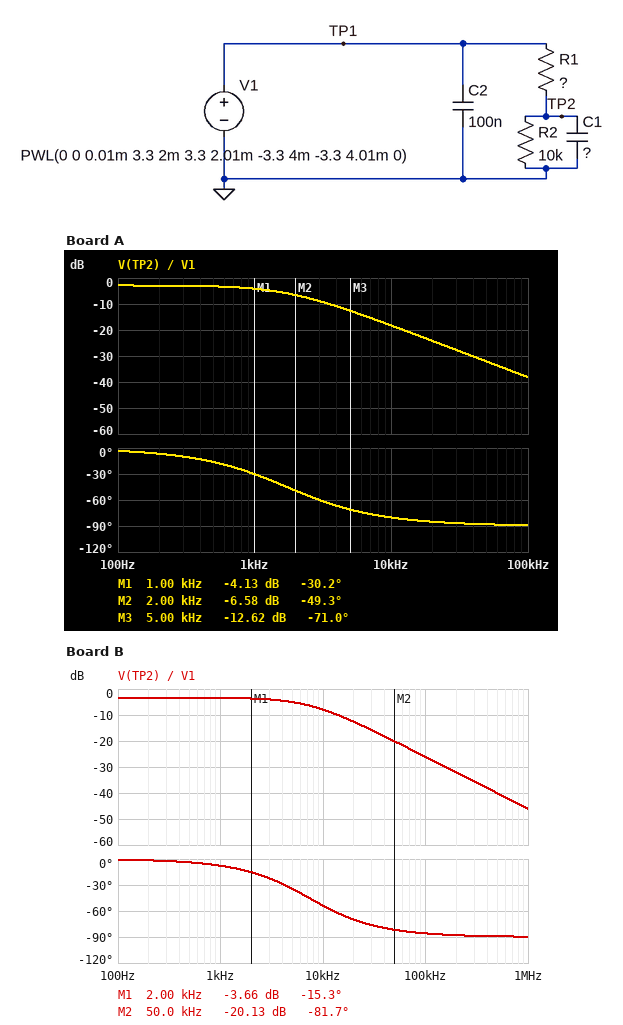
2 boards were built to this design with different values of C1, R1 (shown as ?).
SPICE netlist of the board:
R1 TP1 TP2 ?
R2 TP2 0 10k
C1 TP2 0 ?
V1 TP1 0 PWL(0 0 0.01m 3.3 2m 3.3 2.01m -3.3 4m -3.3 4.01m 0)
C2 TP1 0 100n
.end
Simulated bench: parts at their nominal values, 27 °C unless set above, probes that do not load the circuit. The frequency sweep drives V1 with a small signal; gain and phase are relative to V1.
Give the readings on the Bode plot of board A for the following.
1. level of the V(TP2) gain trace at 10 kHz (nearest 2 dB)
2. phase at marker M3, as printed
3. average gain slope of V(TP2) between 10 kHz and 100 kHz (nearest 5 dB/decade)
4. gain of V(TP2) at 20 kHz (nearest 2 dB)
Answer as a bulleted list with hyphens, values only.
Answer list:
- -18 dB
- -71.0 deg
- -20 dB/decade
- -24 dB
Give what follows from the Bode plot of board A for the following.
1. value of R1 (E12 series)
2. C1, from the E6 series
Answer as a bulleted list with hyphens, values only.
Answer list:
- 3.9 kΩ
- 33 nF
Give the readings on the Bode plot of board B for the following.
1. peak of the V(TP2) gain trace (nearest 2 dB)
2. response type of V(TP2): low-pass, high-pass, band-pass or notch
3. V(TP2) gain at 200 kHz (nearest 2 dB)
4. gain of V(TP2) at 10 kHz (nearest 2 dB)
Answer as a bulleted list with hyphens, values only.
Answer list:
- -4 dB
- low-pass
- -32 dB
- -8 dB
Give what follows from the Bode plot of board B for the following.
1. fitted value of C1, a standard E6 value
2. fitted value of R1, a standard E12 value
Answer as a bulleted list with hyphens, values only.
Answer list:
- 6.8 nF
- 4.7 kΩ
